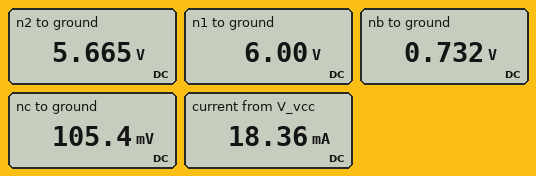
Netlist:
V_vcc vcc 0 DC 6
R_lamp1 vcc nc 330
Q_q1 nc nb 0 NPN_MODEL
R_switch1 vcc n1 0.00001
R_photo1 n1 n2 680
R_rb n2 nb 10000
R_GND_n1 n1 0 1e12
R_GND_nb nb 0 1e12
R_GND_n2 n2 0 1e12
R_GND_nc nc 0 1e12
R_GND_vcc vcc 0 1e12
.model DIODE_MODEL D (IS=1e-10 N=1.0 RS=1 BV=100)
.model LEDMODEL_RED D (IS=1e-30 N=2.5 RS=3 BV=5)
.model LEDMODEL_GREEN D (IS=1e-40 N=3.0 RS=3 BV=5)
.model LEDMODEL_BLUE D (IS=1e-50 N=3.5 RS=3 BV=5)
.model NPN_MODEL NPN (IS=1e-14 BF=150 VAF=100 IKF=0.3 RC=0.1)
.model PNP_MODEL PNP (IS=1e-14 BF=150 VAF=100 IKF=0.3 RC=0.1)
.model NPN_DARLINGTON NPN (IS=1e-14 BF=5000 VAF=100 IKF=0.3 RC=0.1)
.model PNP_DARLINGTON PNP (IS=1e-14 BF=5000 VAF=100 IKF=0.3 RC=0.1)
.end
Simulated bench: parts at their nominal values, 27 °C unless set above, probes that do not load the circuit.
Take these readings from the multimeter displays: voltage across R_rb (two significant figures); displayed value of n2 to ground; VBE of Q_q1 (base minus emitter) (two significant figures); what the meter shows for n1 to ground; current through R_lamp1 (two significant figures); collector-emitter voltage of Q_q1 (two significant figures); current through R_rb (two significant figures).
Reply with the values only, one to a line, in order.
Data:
4.9 V
5.665 V
730 mV
6.00 V
18 mA
110 mV
490 µA
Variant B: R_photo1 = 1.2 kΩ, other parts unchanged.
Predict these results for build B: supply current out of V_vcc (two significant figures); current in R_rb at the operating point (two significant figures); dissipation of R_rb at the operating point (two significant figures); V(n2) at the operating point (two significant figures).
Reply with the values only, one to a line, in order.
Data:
18 mA
470 µA
2.2 mW
5.4 V
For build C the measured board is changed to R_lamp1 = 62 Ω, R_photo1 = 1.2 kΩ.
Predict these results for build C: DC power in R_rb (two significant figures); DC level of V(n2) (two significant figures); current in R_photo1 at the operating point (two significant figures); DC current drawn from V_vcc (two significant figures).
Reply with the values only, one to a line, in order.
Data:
2.2 mW
5.4 V
470 µA
60 mA
